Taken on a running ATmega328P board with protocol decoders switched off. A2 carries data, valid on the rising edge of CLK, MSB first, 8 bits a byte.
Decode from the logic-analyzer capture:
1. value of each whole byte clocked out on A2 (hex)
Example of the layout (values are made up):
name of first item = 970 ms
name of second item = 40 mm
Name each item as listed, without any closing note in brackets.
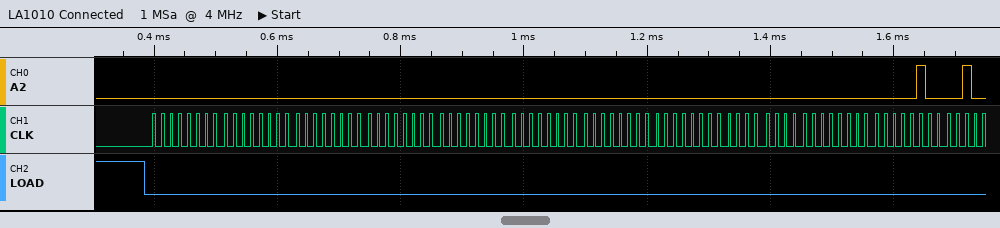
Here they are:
value of each whole byte clocked out on A2 = 00 00 00 00 00 00 00 00 00 00 04
